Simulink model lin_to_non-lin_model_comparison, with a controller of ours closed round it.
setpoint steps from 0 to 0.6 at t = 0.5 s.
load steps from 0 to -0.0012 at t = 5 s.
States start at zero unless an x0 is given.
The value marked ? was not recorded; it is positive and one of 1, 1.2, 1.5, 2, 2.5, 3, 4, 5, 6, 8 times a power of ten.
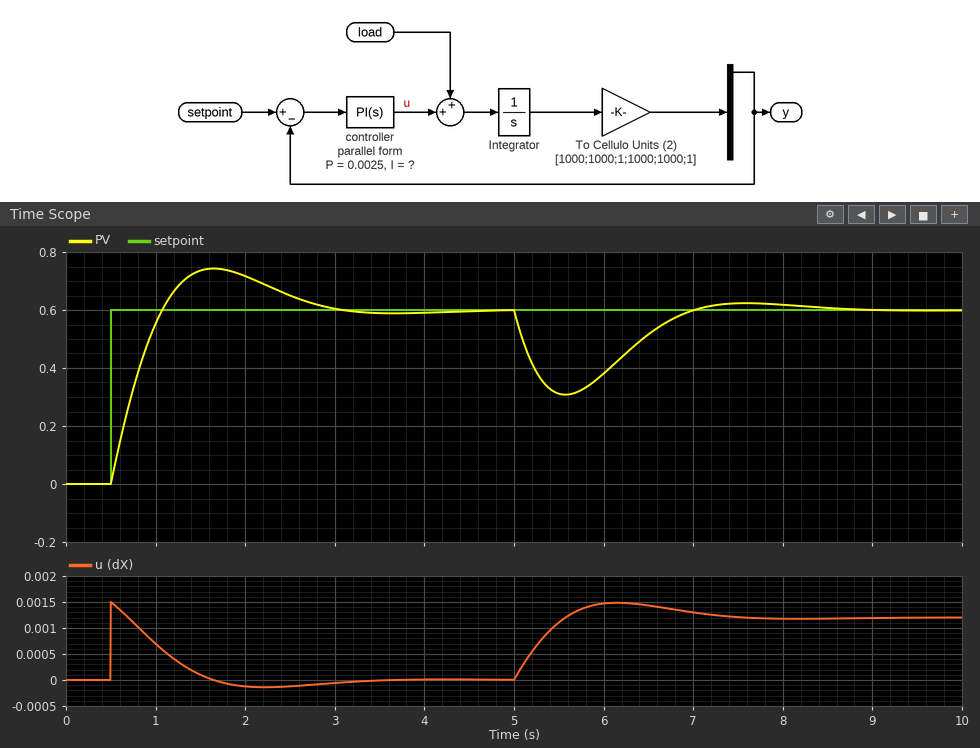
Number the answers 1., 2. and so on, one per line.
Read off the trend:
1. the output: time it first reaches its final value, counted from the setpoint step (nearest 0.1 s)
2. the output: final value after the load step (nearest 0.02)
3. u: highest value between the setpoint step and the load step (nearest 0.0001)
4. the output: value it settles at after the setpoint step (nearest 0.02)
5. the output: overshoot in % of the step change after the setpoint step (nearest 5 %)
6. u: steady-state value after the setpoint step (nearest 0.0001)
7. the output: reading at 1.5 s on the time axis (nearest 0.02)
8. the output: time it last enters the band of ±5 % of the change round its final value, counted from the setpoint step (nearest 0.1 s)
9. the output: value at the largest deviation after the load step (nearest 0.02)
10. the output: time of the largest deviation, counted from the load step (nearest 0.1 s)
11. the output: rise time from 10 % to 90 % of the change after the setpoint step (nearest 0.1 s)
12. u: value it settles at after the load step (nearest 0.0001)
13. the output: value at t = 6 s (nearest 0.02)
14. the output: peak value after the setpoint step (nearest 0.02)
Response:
1. 0.6 s
2. 0.60
3. 0.0015
4. 0.60
5. 25 %
6. 0.0000
7. 0.74
8. 2.2 s
9. 0.30
10. 0.6 s
11. 0.4 s
12. 0.0012
13. 0.38
14. 0.74
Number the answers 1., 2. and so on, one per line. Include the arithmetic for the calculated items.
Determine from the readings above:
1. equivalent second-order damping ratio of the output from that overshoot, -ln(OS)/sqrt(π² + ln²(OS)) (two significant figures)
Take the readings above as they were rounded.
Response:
1. ln(0.25) = -1.386; 1.386 / sqrt(9.870 + 1.922) = 0.40
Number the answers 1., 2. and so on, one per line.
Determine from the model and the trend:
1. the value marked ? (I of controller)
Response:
1. 0.004
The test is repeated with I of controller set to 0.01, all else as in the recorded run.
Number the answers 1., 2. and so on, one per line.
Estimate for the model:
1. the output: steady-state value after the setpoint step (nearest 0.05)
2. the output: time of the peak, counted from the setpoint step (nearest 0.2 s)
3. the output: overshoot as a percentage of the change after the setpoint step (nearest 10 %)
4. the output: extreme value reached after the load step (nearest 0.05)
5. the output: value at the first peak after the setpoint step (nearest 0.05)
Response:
1. 0.60
2. 0.8 s
3. 40 %
4. 0.35
5. 0.80
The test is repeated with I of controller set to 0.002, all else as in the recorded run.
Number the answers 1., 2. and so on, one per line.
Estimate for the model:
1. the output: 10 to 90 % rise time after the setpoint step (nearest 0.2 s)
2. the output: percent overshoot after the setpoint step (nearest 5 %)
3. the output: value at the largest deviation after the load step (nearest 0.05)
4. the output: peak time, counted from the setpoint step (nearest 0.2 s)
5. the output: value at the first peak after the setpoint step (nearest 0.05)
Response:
1. 0.6 s
2. 15 %
3. 0.25
4. 1.4 s
5. 0.70
